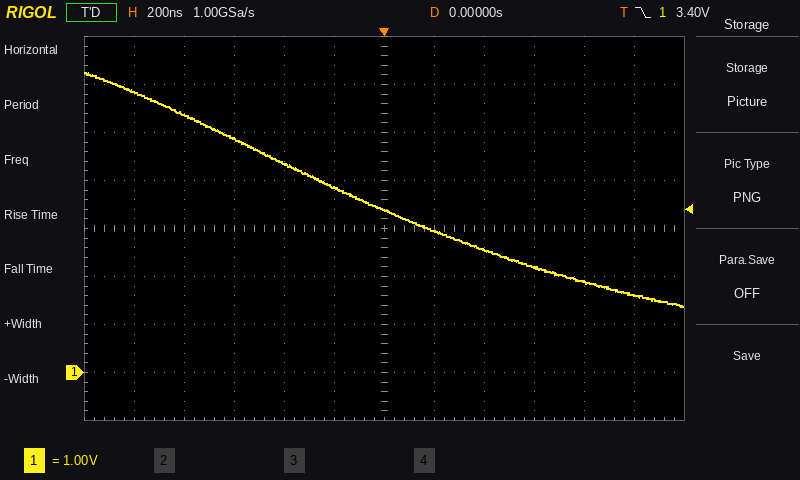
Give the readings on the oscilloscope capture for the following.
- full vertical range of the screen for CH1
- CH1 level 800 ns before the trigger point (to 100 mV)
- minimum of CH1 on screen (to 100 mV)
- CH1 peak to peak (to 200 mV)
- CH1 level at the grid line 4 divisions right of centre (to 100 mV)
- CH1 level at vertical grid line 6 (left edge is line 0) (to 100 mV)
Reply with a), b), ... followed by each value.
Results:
a) 8 V
b) 5.4 V
c) 1.4 V
d) 4.8 V
e) 1.9 V
f) 3.4 V
